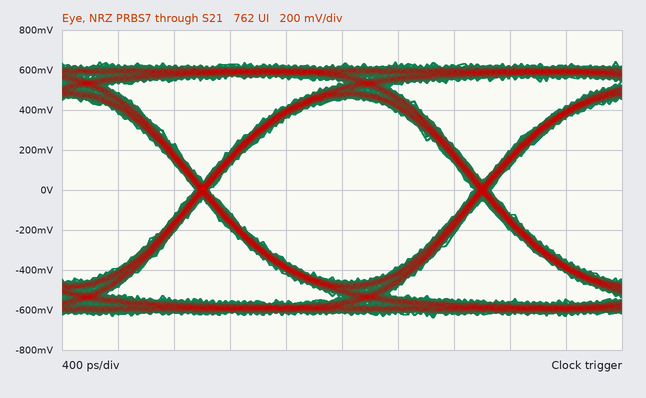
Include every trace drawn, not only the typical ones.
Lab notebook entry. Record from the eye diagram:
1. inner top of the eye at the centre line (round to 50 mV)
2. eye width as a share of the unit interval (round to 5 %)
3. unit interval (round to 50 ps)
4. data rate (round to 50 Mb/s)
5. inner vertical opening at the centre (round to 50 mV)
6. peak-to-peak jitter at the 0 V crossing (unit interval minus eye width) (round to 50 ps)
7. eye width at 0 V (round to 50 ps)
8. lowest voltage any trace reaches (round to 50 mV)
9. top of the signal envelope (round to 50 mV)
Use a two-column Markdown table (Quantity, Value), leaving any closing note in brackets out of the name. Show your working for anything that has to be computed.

| Quantity | Value |
|---|---|
| inner top of the eye at the centre line | 450 mV |
| eye width as a share of the unit interval | 1.90 ns / 2.00 ns ≈ 95 % |
| unit interval | 2.00 ns |
| data rate | 500 Mb/s |
| inner vertical opening at the centre | 900 mV |
| peak-to-peak jitter at the 0 V crossing (unit interval minus eye width) | 100 ps |
| eye width at 0 V | 1.90 ns |
| lowest voltage any trace reaches | -650 mV |
| top of the signal envelope | 650 mV |
